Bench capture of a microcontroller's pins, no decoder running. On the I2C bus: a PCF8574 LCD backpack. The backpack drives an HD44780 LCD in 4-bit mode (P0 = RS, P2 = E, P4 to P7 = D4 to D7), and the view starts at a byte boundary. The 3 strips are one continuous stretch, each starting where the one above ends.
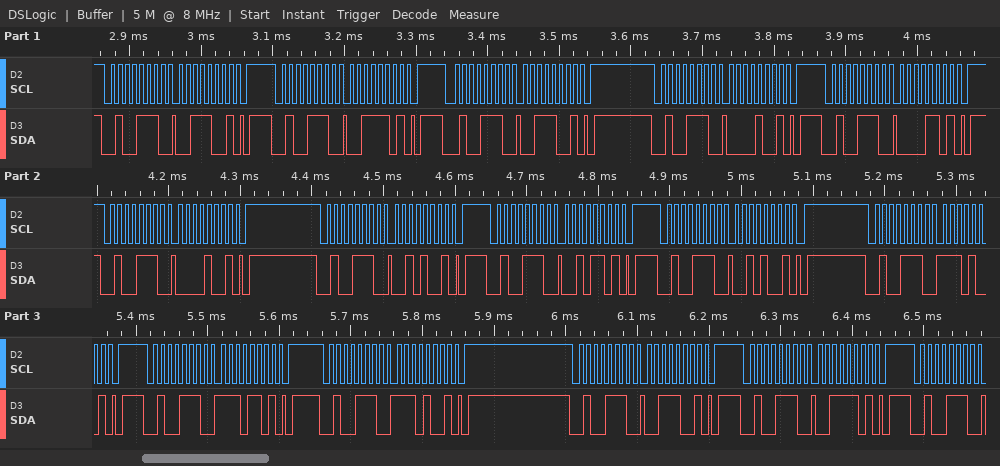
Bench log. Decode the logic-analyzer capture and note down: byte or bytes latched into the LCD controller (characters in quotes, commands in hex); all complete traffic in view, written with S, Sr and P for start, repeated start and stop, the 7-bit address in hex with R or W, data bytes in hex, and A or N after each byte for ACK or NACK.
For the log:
'0' '.'
S 27W A 39 A P S 27W A 3D A P S 27W A 39 A P S 27W A 09 A P S 27W A 0D A P S 27W A 09 A P S 27W A 29 A P S 27W A 2D A P S 27W A 29 A P S 27W A E9 A P S 27W A ED A P S 27W A E9 A P S 27W A 39 A P S 27W A 3D A P S 27W A
